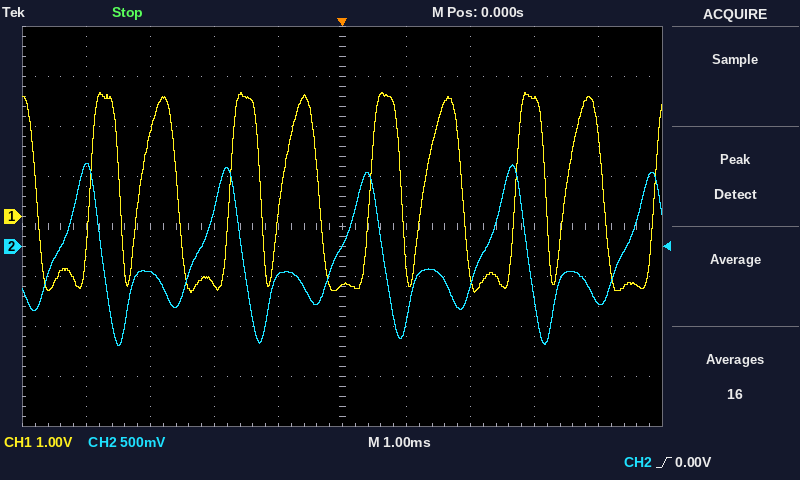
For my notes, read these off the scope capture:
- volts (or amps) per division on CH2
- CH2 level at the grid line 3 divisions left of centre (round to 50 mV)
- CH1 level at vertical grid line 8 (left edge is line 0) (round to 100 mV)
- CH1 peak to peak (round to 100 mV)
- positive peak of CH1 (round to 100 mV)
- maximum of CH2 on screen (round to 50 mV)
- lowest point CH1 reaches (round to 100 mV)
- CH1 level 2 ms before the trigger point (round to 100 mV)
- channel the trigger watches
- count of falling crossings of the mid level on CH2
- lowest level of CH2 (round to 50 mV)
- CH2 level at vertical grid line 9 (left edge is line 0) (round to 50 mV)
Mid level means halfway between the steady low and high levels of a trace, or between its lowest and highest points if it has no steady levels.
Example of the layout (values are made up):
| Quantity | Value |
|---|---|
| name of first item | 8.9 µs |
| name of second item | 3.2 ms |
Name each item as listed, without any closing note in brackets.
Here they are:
| Quantity | Value |
|---|---|
| volts (or amps) per division on CH2 | 500 mV |
| CH2 level at the grid line 3 divisions left of centre | -250 mV |
| CH1 level at vertical grid line 8 (left edge is line 0) | 2.4 V |
| CH1 peak to peak | 4.0 V |
| positive peak of CH1 | 2.5 V |
| maximum of CH2 on screen | 850 mV |
| lowest point CH1 reaches | -1.5 V |
| CH1 level 2 ms before the trigger point | -1.4 V |
| channel the trigger watches | CH2 |
| count of falling crossings of the mid level on CH2 | 4 |
| lowest level of CH2 | -1.00 V |
| CH2 level at vertical grid line 9 (left edge is line 0) | -550 mV |
